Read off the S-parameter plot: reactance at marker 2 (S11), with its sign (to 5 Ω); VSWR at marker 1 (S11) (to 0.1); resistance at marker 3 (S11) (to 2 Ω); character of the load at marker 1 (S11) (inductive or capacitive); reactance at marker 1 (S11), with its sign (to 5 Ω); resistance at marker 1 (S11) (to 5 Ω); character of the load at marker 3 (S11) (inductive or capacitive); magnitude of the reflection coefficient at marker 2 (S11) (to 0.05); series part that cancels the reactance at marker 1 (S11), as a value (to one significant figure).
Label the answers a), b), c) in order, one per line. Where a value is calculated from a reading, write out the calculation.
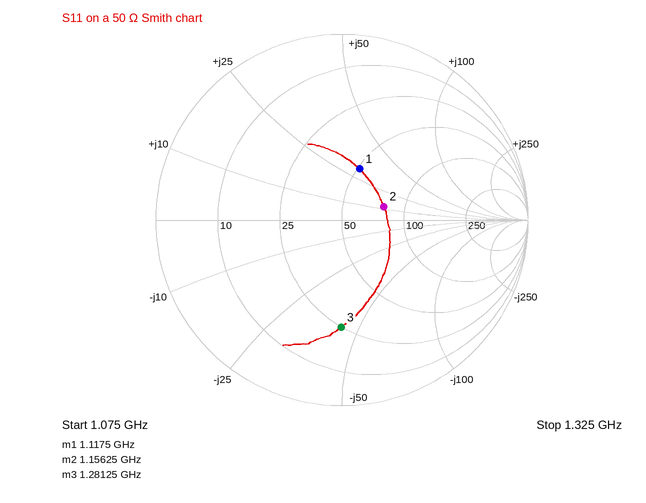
a) +10 Ω
b) 1.8
c) 24 Ω
d) inductive
e) +30 Ω
f) 50 Ω
g) capacitive
h) 0.25
i) C = 1/(2π × 1.1175 GHz × 30 Ω) ≈ 5 pF
